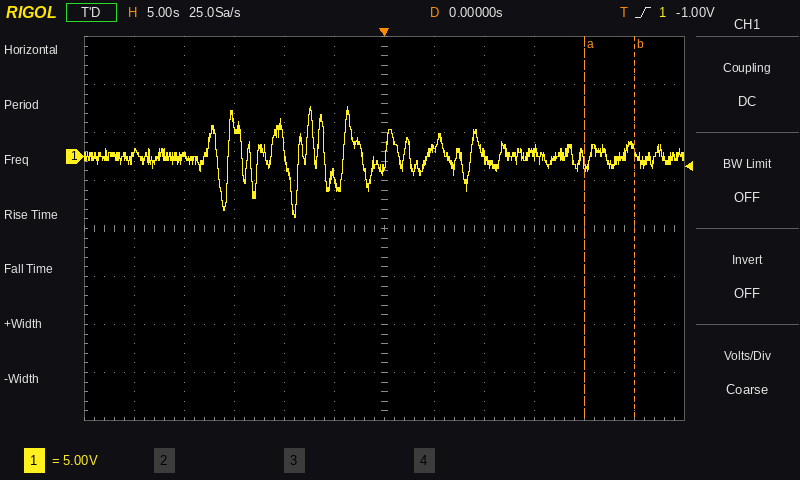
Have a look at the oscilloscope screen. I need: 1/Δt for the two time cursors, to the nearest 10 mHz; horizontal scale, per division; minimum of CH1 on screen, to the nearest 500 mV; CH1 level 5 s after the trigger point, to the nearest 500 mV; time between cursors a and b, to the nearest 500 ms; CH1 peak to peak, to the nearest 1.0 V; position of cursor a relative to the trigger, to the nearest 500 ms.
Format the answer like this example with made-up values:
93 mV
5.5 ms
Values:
200 mHz
5 s
-6.5 V
1.0 V
5.0 s
12.0 V
+20.0 s
